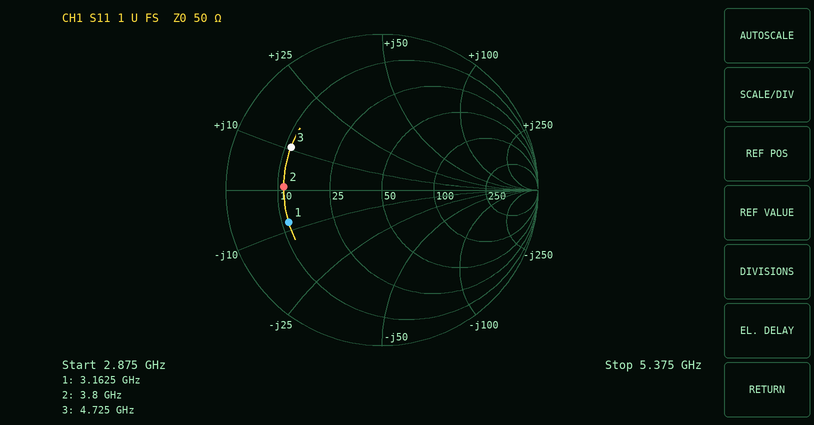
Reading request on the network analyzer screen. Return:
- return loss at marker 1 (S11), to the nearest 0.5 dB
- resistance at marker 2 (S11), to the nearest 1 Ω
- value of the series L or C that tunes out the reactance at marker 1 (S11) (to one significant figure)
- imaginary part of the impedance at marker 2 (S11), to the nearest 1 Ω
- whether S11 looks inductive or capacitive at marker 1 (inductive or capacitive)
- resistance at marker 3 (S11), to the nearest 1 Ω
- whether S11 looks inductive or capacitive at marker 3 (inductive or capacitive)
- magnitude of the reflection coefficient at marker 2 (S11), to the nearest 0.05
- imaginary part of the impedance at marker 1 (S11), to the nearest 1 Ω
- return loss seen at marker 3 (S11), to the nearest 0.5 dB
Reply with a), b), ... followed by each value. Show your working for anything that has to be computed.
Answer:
a) 4.0 dB
b) 11 Ω
c) L = 8 Ω/(2π × 3.1625 GHz) ≈ 403 pH, so 400 pH to one significant figure
d) +1 Ω
e) capacitive
f) 11 Ω
g) inductive
h) 0.65
i) -8 Ω
j) 4.0 dB
